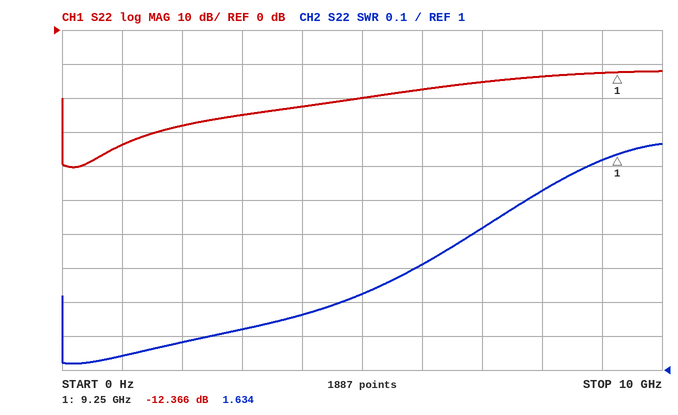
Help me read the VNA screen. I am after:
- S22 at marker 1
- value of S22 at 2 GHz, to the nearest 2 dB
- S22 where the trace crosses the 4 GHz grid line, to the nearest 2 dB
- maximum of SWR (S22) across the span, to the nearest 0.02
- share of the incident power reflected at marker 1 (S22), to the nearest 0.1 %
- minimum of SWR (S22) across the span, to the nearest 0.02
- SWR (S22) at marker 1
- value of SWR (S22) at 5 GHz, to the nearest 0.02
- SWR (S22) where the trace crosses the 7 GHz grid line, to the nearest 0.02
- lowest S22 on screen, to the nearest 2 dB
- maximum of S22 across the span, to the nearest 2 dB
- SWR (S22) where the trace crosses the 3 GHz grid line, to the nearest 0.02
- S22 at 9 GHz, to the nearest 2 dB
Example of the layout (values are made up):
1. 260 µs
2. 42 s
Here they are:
1. -12.366 dB
2. -28 dB
3. -22 dB
4. 1.66
5. 5.8 %
6. 1.02
7. 1.634
8. 1.22
9. 1.42
10. -40 dB
11. -12 dB
12. 1.12
13. -12 dB
